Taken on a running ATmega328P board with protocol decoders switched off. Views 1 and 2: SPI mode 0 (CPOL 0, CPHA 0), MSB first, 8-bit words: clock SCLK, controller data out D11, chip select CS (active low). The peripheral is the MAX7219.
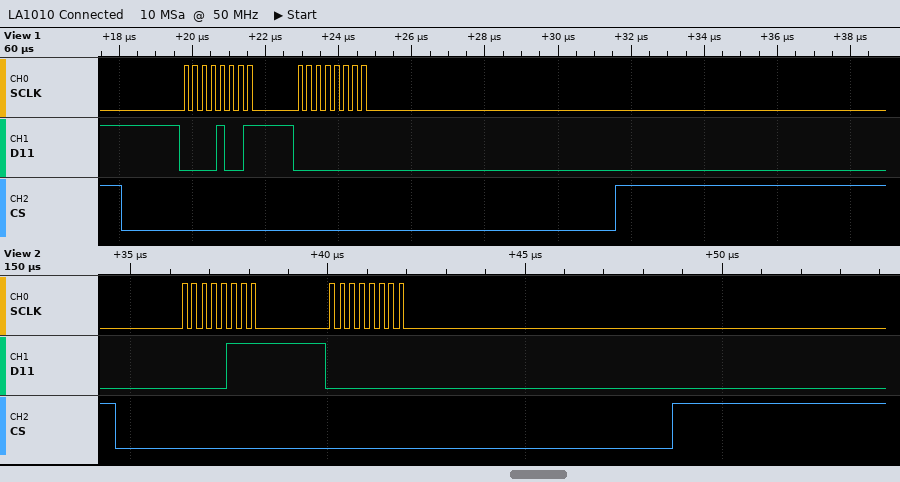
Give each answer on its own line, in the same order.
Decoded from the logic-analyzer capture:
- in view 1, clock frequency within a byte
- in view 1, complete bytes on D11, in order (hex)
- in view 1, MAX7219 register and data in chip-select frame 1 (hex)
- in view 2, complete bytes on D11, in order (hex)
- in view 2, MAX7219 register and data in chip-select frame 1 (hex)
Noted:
4 MHz
09 00
register 0x9, data 0x00
07 00
register 0x7, data 0x00
